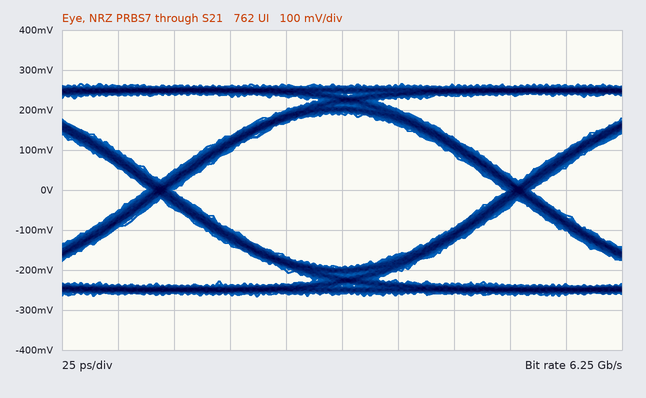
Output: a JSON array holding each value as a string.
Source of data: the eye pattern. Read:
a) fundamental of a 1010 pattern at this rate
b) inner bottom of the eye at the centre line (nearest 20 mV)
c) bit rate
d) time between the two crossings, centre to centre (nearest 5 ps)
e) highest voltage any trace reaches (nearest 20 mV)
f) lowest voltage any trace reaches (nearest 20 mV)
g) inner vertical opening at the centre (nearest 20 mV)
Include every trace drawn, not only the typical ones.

["3.125 GHz", "-200 mV", "6.25 Gb/s", "160 ps", "260 mV", "-260 mV", "380 mV"]
